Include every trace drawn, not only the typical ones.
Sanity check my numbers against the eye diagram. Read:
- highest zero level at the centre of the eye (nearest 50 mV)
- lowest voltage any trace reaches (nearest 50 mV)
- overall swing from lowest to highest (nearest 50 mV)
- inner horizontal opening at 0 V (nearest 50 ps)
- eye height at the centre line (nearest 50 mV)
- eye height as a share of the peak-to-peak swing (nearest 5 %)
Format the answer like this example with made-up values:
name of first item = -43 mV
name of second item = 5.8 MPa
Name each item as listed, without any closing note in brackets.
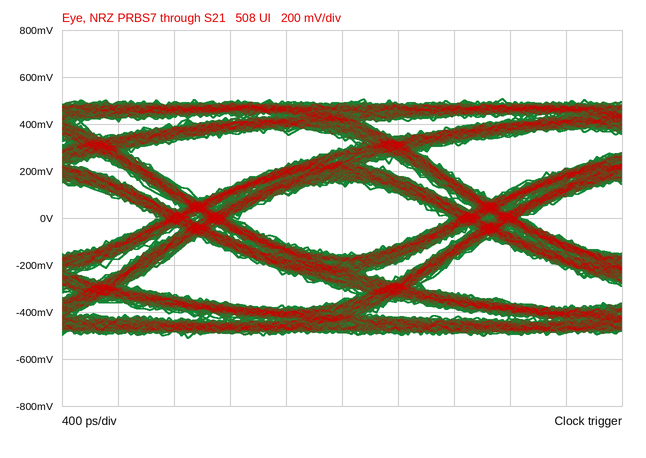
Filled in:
highest zero level at the centre of the eye = -150 mV
lowest voltage any trace reaches = -500 mV
overall swing from lowest to highest = 1.00 V
inner horizontal opening at 0 V = 1.50 ns
eye height at the centre line = 300 mV
eye height as a share of the peak-to-peak swing = 30 %
